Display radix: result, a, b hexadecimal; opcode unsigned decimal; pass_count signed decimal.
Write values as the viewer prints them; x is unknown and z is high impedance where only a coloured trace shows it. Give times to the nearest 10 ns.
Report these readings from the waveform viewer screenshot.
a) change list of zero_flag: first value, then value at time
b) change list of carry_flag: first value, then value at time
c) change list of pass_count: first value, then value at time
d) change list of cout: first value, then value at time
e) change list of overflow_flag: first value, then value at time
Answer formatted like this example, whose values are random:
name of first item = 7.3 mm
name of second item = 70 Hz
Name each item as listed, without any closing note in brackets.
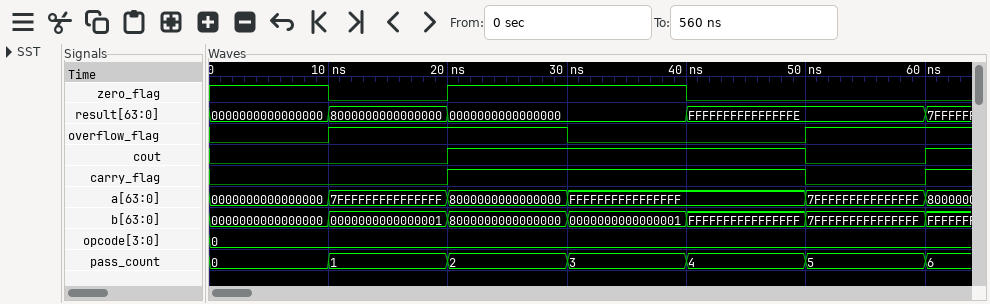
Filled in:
change list of zero_flag: first value, then value at time = 1, 0 at 10 ns, 1 at 20 ns, 0 at 40 ns
change list of carry_flag: first value, then value at time = 0, 1 at 20 ns, 0 at 50 ns, 1 at 60 ns
change list of pass_count: first value, then value at time = 0, 1 at 10 ns, 2 at 20 ns, 3 at 30 ns, 4 at 40 ns, 5 at 50 ns, 6 at 60 ns
change list of cout: first value, then value at time = 0, 1 at 20 ns, 0 at 50 ns, 1 at 60 ns
change list of overflow_flag: first value, then value at time = 0, 1 at 10 ns, 0 at 30 ns, 1 at 50 ns
